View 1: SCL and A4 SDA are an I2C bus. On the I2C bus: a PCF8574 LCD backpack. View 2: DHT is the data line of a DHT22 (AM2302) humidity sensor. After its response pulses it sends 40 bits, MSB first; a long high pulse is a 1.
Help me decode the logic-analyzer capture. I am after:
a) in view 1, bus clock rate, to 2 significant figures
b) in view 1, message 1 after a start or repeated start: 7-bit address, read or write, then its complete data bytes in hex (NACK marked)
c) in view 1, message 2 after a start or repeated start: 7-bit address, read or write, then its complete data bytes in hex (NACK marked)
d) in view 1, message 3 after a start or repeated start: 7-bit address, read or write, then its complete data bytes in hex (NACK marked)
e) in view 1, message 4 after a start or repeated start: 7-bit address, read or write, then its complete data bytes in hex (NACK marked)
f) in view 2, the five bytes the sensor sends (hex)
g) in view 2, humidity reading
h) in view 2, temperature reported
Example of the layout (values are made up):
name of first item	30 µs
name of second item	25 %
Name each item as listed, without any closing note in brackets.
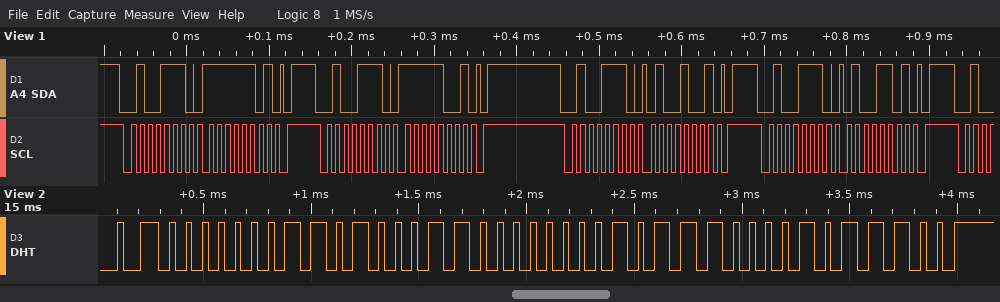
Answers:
in view 1, bus clock rate, to 2 significant figures	100 kHz
in view 1, message 1 after a start or repeated start: 7-bit address, read or write, then its complete data bytes in hex	0x27 write: FD
in view 1, message 2 after a start or repeated start: 7-bit address, read or write, then its complete data bytes in hex	0x27 write: F9
in view 1, message 3 after a start or repeated start: 7-bit address, read or write, then its complete data bytes in hex	0x27 write: 49
in view 1, message 4 after a start or repeated start: 7-bit address, read or write, then its complete data bytes in hex	0x27 write: 4D
in view 2, the five bytes the sensor sends	01 A3 00 B8 5C
in view 2, humidity reading	41.9 %
in view 2, temperature reported	18.4 °C
